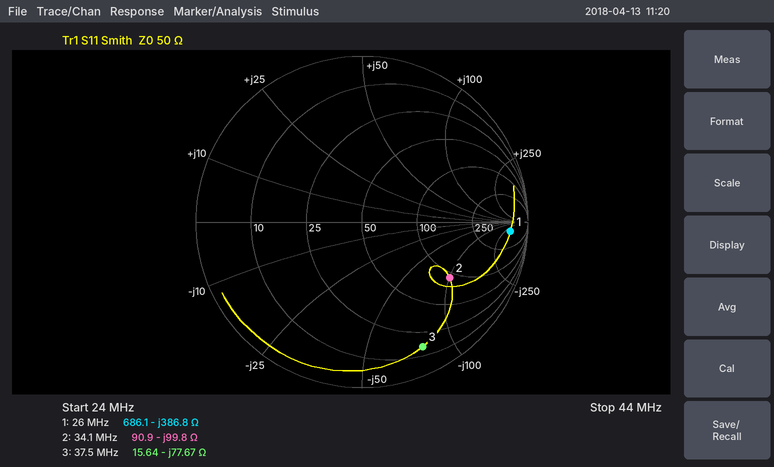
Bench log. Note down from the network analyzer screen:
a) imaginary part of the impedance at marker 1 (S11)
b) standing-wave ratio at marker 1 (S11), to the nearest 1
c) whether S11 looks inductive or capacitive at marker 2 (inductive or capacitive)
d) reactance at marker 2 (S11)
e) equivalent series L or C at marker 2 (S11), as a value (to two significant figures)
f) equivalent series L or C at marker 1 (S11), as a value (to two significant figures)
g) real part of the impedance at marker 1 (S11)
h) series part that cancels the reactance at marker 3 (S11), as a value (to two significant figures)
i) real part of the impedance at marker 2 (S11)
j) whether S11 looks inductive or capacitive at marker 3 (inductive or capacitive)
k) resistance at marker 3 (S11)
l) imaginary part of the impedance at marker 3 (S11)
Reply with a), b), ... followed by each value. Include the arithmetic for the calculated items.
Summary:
a) -386.8 Ω
b) 18
c) capacitive
d) -99.8 Ω
e) C = 1/(2π × 34.1 MHz × 99.8 Ω) ≈ 47 pF
f) C = 1/(2π × 26 MHz × 386.8 Ω) ≈ 16 pF
g) 686.1 Ω
h) L = 77.67 Ω/(2π × 37.5 MHz) ≈ 330 nH
i) 90.9 Ω
j) capacitive
k) 15.64 Ω
l) -77.67 Ω
